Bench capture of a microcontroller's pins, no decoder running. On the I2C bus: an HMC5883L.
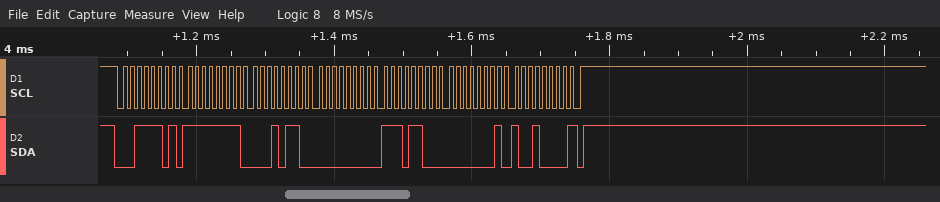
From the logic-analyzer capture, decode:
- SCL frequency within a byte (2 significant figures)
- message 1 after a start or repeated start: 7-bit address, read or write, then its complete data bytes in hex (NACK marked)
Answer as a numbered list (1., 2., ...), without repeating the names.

1. 100 kHz
2. 0x1E read: FF 16 00 EC 01 90 NACK
